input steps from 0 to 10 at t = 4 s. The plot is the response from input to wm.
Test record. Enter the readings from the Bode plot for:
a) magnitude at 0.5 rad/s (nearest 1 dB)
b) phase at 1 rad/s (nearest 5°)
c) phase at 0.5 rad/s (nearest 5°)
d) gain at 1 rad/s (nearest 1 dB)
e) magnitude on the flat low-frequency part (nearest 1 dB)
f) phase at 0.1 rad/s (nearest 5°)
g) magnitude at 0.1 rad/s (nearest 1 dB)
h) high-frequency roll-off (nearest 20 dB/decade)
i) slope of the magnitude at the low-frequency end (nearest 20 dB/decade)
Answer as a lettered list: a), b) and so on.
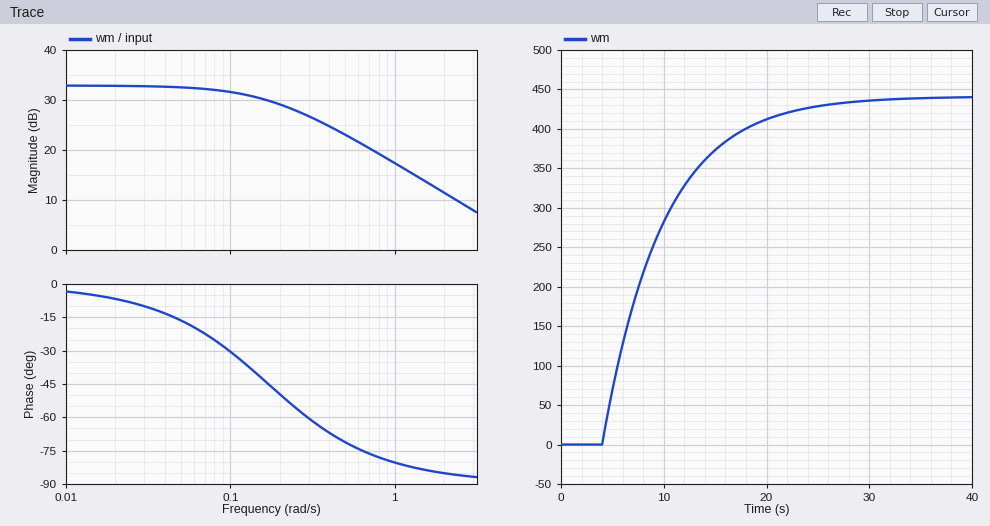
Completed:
a) 23 dB
b) -80°
c) -70°
d) 17 dB
e) 33 dB
f) -30°
g) 32 dB
h) -20 dB/decade
i) 0 dB/decade
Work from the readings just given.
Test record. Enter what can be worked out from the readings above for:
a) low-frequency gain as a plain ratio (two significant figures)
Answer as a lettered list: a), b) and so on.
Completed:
a) 45
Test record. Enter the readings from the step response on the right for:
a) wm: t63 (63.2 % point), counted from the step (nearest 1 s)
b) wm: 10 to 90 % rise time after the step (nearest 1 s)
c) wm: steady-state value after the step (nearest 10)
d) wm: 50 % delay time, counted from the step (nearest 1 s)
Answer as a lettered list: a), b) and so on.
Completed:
a) 6 s
b) 13 s
c) 440
d) 4 s
